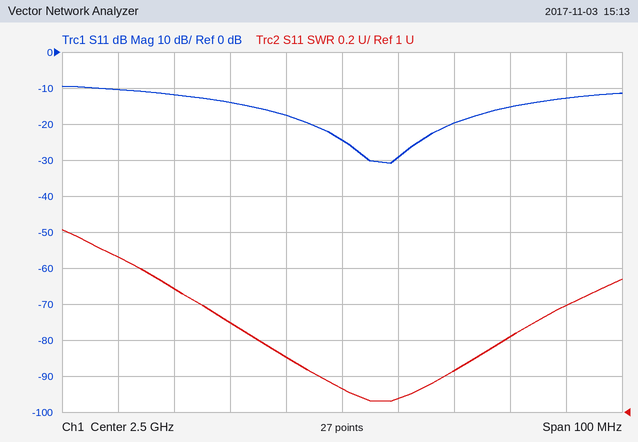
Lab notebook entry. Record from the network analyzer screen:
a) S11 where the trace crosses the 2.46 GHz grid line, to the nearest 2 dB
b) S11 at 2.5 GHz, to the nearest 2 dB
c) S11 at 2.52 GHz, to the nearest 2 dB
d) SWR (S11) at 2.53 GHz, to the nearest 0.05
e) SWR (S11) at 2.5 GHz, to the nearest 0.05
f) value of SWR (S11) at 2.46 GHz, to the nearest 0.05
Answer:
-10 dB
-24 dB
-20 dB
1.40
1.15
1.85
